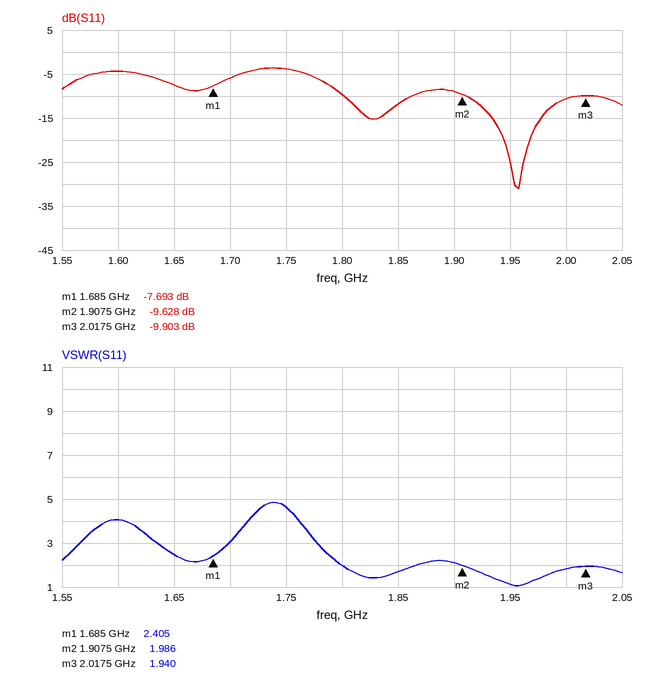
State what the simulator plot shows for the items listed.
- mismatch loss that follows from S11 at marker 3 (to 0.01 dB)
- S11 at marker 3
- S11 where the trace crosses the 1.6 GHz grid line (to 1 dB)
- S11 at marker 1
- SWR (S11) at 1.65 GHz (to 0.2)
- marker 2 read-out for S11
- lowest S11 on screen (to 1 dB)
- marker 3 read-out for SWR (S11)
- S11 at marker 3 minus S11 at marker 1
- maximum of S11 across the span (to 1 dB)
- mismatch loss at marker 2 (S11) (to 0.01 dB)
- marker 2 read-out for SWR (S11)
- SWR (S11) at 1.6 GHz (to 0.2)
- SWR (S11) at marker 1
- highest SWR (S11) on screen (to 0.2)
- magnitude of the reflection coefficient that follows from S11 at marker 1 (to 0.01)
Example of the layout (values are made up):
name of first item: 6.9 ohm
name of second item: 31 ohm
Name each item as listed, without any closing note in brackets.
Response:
mismatch loss that follows from S11 at marker 3: 0.47 dB
S11 at marker 3: -9.903 dB
S11 where the trace crosses the 1.6 GHz grid line: -4 dB
S11 at marker 1: -7.693 dB
SWR (S11) at 1.65 GHz: 2.4
marker 2 read-out for S11: -9.628 dB
lowest S11 on screen: -31 dB
marker 3 read-out for SWR: 1.940
S11 at marker 3 minus S11 at marker 1: -2.210 dB
maximum of S11 across the span: -4 dB
mismatch loss at marker 2 (S11): 0.50 dB
marker 2 read-out for SWR: 1.986
SWR (S11) at 1.6 GHz: 4.0
SWR (S11) at marker 1: 2.405
highest SWR (S11) on screen: 4.8
magnitude of the reflection coefficient that follows from S11 at marker 1: 0.41
